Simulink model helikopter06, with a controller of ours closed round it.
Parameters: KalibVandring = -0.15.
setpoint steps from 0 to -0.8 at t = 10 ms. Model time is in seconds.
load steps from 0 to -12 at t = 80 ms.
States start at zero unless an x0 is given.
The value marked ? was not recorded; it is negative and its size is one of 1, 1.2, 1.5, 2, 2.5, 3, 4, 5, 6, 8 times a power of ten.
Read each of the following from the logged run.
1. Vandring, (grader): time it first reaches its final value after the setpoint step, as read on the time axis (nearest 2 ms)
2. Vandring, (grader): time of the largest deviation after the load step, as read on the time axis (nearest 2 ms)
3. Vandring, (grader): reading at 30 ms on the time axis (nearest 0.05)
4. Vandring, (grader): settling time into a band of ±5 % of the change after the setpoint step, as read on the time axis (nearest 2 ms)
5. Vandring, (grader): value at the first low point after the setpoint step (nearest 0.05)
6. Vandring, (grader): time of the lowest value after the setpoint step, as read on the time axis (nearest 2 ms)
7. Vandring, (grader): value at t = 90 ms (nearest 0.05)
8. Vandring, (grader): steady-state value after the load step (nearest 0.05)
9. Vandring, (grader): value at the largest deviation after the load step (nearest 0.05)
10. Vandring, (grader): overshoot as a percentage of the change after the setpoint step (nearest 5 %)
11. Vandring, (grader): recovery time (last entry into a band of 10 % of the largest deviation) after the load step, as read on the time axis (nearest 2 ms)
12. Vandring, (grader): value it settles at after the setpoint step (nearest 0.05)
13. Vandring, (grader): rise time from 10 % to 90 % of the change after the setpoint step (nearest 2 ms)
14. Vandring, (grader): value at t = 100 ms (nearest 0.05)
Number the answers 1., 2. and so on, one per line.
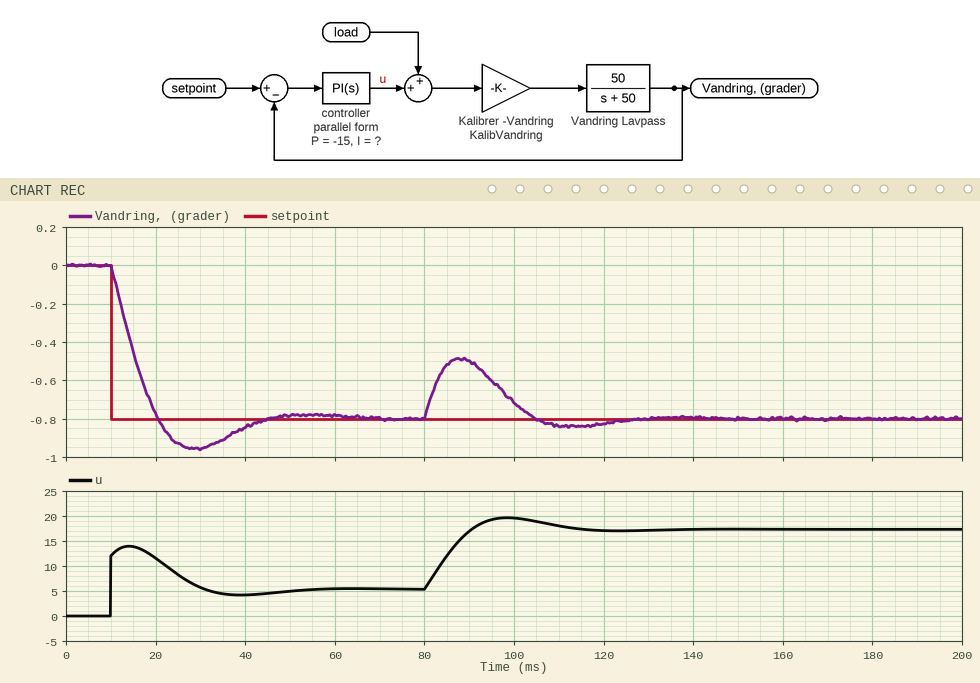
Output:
1. 20 ms
2. 88 ms
3. -0.95
4. 40 ms
5. -0.95
6. 28 ms
7. -0.50
8. -0.80
9. -0.50
10. 20 %
11. 118 ms
12. -0.80
13. 8 ms
14. -0.70
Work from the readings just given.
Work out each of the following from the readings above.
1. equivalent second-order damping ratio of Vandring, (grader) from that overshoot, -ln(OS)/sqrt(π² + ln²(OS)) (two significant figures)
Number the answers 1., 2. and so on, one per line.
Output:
1. 0.46
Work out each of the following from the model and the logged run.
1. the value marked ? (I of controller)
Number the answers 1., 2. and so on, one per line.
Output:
1. -3000
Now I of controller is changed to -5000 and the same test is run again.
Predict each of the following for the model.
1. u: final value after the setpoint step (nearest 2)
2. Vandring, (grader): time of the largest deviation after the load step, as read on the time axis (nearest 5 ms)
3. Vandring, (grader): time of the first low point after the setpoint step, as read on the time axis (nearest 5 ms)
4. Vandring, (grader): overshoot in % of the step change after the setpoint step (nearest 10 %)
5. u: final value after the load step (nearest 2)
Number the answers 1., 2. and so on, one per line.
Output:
1. 6
2. 85 ms
3. 25 ms
4. 30 %
5. 18
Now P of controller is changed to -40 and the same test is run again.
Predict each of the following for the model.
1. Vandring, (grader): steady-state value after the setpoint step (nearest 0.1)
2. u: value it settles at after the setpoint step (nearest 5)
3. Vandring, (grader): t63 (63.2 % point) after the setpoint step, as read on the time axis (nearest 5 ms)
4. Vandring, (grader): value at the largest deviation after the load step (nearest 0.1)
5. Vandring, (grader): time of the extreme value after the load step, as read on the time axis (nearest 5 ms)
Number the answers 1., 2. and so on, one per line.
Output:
1. -0.8
2. 5
3. 15 ms
4. -0.6
5. 85 ms
